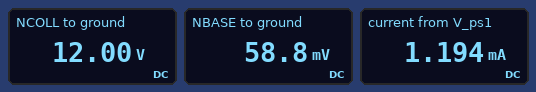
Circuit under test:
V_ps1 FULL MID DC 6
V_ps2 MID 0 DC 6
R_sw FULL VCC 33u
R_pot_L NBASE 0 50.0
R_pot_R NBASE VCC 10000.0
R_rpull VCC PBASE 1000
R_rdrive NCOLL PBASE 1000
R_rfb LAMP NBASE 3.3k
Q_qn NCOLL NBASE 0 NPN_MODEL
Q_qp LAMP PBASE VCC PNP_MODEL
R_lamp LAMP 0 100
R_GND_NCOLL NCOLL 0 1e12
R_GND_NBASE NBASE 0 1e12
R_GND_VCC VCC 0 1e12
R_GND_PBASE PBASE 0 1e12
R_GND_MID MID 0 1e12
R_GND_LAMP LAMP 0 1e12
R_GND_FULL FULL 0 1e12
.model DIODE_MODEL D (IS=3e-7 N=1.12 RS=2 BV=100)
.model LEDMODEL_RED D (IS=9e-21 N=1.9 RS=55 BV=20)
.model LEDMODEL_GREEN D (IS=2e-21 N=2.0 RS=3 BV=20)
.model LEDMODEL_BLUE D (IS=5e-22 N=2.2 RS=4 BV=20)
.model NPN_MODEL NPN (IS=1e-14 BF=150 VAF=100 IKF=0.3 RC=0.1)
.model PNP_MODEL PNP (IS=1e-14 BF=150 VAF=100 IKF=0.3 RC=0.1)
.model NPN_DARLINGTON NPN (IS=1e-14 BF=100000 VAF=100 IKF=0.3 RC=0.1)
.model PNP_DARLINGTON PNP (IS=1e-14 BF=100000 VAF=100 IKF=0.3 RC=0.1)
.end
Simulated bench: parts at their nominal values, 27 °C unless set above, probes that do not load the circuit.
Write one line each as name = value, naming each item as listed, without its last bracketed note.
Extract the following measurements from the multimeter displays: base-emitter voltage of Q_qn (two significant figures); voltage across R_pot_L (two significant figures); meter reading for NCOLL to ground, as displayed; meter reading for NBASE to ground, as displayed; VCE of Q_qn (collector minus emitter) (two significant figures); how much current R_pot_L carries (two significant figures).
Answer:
base-emitter voltage of Q_qn = 59 mV
voltage across R_pot_L = 59 mV
meter reading for NCOLL to ground, as displayed = 12.00 V
meter reading for NBASE to ground, as displayed = 58.8 mV
VCE of Q_qn (collector minus emitter) = 12 V
how much current R_pot_L carries = 1.2 mA
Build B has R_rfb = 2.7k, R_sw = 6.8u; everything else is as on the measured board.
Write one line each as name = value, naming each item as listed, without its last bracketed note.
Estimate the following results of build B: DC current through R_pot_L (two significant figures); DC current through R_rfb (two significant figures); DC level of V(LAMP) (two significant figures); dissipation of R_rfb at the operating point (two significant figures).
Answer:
DC current through R_pot_L = 1.2 mA
DC current through R_rfb = 21 µA
DC level of V(LAMP) = 2.1 mV
dissipation of R_rfb at the operating point = 1.2 µW
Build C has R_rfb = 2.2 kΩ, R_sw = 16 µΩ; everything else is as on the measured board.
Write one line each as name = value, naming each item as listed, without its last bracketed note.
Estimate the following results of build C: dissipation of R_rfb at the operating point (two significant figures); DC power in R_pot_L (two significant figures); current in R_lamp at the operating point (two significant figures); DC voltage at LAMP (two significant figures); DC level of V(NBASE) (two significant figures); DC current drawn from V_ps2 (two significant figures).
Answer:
dissipation of R_rfb at the operating point = 1.4 µW
DC power in R_pot_L = 68 µW
current in R_lamp at the operating point = 25 µA
DC voltage at LAMP = 2.5 mV
DC level of V(NBASE) = 58 mV
DC current drawn from V_ps2 = 1.2 mA
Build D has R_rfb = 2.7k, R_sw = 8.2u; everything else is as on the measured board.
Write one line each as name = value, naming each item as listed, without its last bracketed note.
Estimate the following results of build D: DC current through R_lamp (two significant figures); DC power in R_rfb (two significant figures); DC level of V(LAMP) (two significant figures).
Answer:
DC current through R_lamp = 21 µA
DC power in R_rfb = 1.2 µW
DC level of V(LAMP) = 2.1 mV
